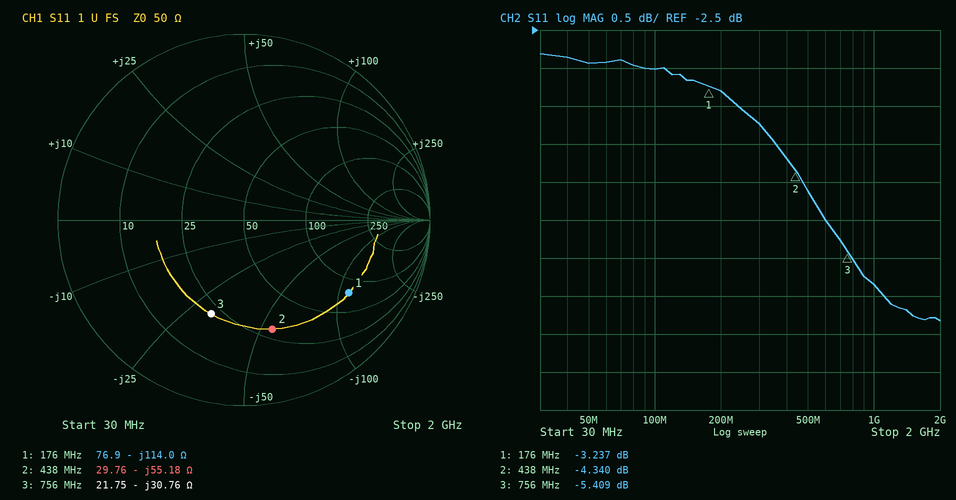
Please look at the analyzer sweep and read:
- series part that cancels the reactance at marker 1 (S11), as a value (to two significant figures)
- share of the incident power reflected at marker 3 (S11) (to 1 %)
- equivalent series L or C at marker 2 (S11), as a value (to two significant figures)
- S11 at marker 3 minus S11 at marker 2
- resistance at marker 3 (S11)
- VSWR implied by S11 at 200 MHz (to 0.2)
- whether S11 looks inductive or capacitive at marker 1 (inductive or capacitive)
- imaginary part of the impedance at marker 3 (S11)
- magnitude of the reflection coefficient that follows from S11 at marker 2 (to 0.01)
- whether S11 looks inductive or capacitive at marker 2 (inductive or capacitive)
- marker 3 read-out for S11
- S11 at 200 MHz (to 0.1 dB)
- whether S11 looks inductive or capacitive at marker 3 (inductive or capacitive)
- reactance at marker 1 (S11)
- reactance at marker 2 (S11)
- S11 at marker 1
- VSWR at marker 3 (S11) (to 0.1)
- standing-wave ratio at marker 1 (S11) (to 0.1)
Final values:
100 nH
29 %
6.6 pF
-1.069 dB
21.75 Ω
5.4
capacitive
-30.76 Ω
0.61
capacitive
-5.409 dB
-3.3 dB
capacitive
-114.0 Ω
-55.18 Ω
-3.237 dB
3.3
5.4
